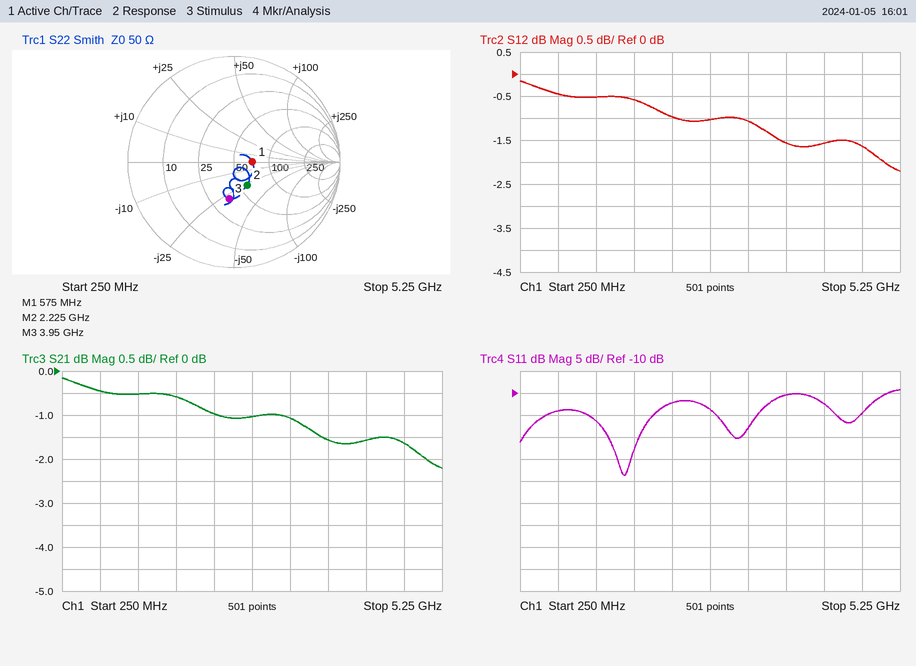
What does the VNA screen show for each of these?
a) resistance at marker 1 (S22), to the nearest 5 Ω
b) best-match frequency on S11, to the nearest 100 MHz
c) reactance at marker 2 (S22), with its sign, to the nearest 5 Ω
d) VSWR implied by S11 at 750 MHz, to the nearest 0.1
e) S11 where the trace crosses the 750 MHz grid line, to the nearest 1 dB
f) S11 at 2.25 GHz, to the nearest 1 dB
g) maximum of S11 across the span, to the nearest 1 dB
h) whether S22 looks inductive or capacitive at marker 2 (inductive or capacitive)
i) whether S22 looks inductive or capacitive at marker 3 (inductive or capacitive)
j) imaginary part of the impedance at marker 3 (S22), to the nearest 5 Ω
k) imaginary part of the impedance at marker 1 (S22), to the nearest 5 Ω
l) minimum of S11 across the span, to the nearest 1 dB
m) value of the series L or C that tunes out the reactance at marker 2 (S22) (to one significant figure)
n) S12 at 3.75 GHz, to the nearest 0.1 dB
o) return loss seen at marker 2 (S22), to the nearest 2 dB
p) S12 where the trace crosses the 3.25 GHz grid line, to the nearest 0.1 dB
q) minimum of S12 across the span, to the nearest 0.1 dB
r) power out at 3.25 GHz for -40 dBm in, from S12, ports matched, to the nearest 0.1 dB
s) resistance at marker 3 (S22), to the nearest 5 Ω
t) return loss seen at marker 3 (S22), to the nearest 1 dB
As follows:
70 Ω
1.6 GHz
-25 Ω
1.5
-14 dB
-12 dB
-9 dB
capacitive
capacitive
-30 Ω
0 Ω
-29 dB
2 nH
-1.6 dB
12 dB
-1.1 dB
-2.2 dB
-41.1 dBm
35 Ω
9 dB
